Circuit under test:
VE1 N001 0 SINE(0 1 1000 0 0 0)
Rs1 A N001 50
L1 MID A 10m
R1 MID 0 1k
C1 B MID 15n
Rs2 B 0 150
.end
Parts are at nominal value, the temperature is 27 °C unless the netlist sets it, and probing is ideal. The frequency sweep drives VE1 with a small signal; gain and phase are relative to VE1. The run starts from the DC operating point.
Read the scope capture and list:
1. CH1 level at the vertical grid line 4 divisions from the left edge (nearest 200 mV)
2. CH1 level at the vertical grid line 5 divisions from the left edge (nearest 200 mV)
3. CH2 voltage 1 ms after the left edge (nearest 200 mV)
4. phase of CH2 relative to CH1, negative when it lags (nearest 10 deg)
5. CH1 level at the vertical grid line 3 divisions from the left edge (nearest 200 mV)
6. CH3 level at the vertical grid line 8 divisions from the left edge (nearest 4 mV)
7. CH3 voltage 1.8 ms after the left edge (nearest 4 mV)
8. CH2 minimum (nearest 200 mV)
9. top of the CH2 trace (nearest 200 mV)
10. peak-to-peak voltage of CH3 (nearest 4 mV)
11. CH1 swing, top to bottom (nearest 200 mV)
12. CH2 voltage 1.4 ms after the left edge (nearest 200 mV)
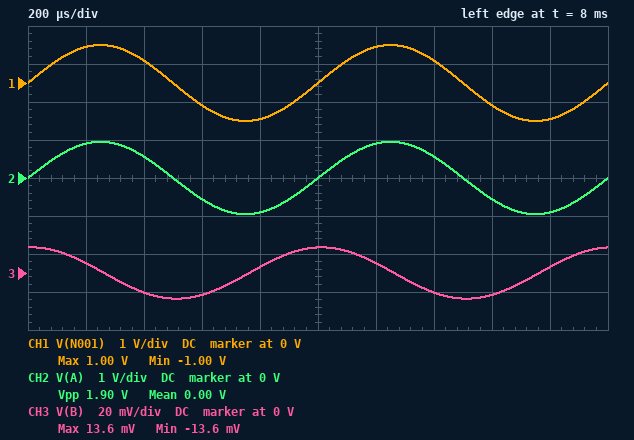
-1.0 V
0 V
0 V
0 deg
-600 mV
-12 mV
4 mV
-1.0 V
1.0 V
28 mV
2.0 V
600 mV
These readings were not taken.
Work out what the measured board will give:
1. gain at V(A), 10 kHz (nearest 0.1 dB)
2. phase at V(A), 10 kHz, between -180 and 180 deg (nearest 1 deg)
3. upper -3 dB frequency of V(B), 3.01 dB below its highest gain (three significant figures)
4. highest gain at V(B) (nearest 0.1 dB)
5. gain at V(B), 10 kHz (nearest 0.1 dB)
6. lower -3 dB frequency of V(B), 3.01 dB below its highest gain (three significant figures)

-0.7 dB
2 deg
19.9 kHz
-15.3 dB
-16.1 dB
7.76 kHz
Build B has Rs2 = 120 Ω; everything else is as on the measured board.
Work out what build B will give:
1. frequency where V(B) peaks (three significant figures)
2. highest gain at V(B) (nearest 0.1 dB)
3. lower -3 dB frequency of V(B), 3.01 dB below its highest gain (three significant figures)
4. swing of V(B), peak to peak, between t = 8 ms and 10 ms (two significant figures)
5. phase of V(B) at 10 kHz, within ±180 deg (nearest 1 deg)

12.6 kHz
-16.9 dB
7.95 kHz
22 mV
26 deg
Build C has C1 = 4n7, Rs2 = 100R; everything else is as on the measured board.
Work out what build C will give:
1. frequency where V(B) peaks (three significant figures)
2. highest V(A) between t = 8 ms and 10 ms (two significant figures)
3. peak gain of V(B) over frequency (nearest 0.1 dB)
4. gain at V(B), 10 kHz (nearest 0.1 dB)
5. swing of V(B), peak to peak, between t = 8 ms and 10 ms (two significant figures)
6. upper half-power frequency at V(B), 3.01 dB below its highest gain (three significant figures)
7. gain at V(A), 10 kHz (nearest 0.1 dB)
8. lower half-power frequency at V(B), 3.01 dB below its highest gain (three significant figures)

22.7 kHz
950 mV
-27.2 dB
-31.3 dB
5.6 mV
44.6 kHz
-0.4 dB
11.5 kHz
